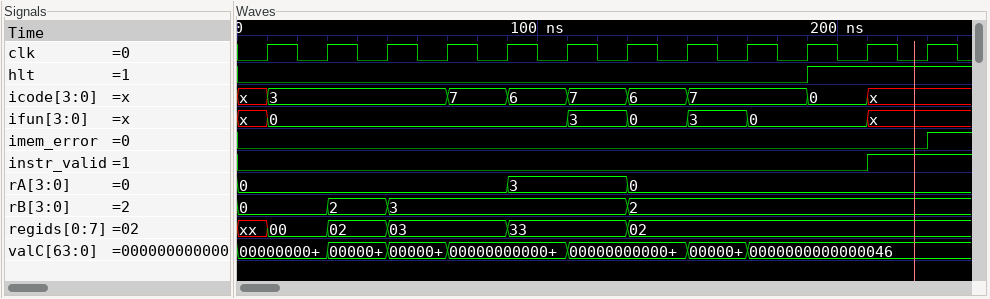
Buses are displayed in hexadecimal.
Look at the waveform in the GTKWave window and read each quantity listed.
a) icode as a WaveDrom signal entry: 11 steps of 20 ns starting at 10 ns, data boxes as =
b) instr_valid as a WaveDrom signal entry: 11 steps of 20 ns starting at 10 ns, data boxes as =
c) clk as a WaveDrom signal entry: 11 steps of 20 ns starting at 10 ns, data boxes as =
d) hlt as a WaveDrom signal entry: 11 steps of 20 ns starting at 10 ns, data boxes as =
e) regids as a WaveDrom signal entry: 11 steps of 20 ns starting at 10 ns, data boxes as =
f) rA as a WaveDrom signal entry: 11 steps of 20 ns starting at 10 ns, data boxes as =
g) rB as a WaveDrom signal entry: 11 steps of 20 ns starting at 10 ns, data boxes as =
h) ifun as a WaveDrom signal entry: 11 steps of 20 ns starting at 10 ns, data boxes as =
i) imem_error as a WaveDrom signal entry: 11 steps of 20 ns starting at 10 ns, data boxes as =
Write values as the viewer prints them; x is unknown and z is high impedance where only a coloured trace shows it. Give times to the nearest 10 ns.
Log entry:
{name: 'icode', wave: '=..=====.=x', data: '3 7 6 7 6 7 0'}
{name: 'instr_valid', wave: '0.........1'}
{name: 'clk', wave: 'p..........'}
{name: 'hlt', wave: '0........1.'}
{name: 'regids', wave: '===.=.=....', data: '00 02 03 33 02'}
{name: 'rA', wave: '=...=.=....', data: '0 3 0'}
{name: 'rB', wave: '===...=....', data: '0 2 3 2'}
{name: 'ifun', wave: '=....====.x', data: '0 3 0 3 0'}
{name: 'imem_error', wave: '0..........'}
